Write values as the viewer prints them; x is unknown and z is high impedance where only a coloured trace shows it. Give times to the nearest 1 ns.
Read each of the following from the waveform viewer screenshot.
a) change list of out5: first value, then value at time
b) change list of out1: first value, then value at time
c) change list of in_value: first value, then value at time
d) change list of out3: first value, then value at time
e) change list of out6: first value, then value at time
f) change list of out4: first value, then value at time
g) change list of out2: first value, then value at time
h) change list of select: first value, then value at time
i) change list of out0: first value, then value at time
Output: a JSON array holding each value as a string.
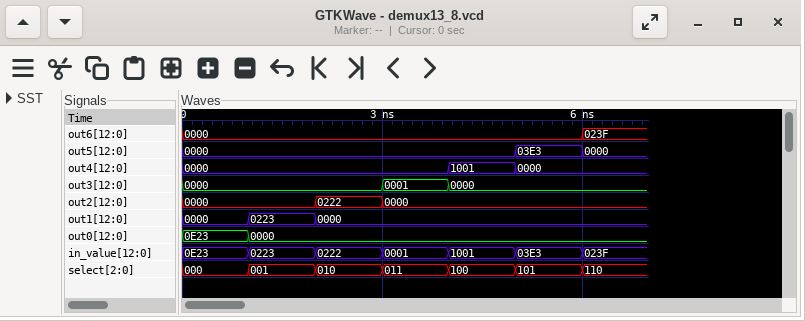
["0000, 03E3 at 5 ns, 0000 at 6 ns", "0000, 0223 at 1 ns, 0000 at 2 ns", "0E23, 0223 at 1 ns, 0222 at 2 ns, 0001 at 3 ns, 1001 at 4 ns, 03E3 at 5 ns, 023F at 6 ns", "0000, 0001 at 3 ns, 0000 at 4 ns", "0000, 023F at 6 ns", "0000, 1001 at 4 ns, 0000 at 5 ns", "0000, 0222 at 2 ns, 0000 at 3 ns", "000, 001 at 1 ns, 010 at 2 ns, 011 at 3 ns, 100 at 4 ns, 101 at 5 ns, 110 at 6 ns", "0E23, 0000 at 1 ns"]
